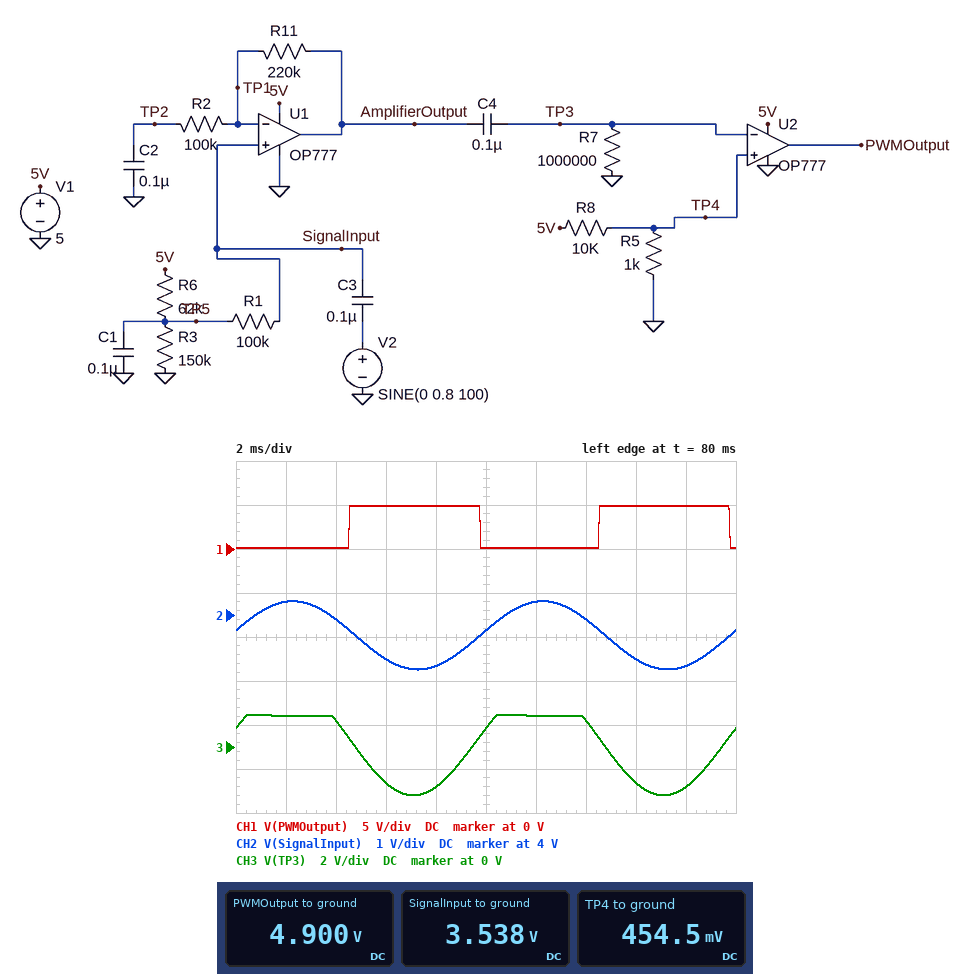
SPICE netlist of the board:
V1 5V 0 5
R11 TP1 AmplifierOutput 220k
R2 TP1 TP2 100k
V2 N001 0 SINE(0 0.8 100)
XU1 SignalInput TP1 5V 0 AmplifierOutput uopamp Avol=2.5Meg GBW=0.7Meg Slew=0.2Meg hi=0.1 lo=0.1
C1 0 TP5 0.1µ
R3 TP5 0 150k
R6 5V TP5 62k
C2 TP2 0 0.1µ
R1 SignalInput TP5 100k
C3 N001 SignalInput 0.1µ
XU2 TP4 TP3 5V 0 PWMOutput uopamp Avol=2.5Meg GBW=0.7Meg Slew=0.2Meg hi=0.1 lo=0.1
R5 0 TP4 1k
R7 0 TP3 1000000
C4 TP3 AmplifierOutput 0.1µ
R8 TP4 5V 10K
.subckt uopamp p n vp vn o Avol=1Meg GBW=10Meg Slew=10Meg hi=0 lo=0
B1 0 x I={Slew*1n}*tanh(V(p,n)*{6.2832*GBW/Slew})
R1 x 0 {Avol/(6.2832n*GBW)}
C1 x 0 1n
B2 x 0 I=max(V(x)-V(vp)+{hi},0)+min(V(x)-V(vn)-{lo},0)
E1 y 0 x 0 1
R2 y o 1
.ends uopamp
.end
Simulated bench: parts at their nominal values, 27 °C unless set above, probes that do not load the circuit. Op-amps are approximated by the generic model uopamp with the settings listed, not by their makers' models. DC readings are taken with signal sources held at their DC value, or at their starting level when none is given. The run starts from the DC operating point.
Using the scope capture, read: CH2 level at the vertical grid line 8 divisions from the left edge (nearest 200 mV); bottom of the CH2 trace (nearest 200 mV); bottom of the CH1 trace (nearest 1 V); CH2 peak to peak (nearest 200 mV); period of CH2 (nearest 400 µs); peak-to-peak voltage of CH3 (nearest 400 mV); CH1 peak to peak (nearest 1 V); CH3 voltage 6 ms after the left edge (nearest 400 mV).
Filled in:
3.0 V
2.8 V
0 V
1.6 V
10.0 ms
3.6 V
5 V
-1.6 V
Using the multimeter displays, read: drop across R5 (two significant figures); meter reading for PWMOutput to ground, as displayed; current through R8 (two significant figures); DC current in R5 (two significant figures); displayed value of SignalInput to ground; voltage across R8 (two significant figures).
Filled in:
450 mV
4.900 V
450 µA
450 µA
3.538 V
4.5 V
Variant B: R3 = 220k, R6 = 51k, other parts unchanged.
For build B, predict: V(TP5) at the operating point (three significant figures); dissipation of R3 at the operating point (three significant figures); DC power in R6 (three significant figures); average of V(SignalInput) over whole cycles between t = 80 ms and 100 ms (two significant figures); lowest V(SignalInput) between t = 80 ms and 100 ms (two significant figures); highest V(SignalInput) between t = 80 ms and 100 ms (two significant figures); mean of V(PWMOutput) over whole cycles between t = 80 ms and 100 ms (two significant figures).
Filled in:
4.06 V
74.9 µW
17.4 µW
4.1 V
3.3 V
4.8 V
2.5 V
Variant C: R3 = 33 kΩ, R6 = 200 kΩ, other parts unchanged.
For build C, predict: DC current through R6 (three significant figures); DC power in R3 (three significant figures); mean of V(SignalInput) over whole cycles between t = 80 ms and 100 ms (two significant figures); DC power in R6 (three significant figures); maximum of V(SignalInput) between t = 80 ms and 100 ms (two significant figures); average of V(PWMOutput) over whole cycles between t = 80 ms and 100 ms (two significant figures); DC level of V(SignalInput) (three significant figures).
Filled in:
21.5 µA
15.2 µW
710 mV
92.1 µW
1.5 V
3.2 V
708 mV
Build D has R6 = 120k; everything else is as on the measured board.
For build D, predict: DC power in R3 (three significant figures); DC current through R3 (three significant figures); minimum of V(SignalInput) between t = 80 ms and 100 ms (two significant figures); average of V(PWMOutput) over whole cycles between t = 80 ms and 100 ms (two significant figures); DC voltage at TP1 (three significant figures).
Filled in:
51.4 µW
18.5 µA
2.0 V
2.8 V
2.78 V
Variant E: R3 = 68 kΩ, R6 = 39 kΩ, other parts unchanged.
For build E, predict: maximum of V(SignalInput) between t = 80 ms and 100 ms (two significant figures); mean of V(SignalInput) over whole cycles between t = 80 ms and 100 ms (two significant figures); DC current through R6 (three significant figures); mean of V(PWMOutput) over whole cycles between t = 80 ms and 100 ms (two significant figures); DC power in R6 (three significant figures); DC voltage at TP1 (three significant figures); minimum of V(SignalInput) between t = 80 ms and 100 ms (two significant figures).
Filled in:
4.0 V
3.2 V
46.7 µA
2.7 V
85.2 µW
3.18 V
2.4 V
